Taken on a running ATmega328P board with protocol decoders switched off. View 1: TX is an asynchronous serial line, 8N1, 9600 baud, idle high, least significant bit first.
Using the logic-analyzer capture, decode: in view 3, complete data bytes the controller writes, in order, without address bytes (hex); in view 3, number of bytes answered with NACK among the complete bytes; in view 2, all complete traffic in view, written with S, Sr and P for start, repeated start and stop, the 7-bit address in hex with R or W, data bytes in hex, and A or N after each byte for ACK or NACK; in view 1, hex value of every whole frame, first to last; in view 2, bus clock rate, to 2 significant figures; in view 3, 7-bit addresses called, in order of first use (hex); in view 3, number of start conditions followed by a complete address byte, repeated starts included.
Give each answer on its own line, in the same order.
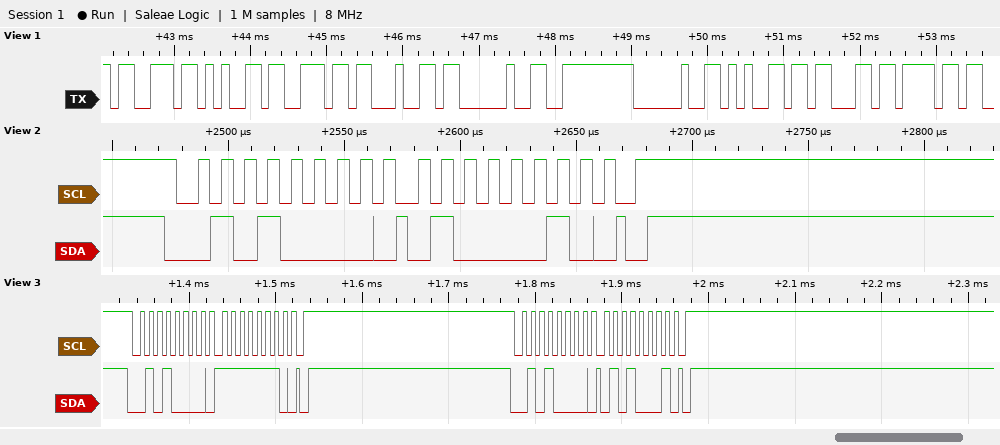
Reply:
FE 51
0
S 28W A 42 A P
73 65 6E 64 20 FE 20 65 63 6F
100 kHz
0x28
2
